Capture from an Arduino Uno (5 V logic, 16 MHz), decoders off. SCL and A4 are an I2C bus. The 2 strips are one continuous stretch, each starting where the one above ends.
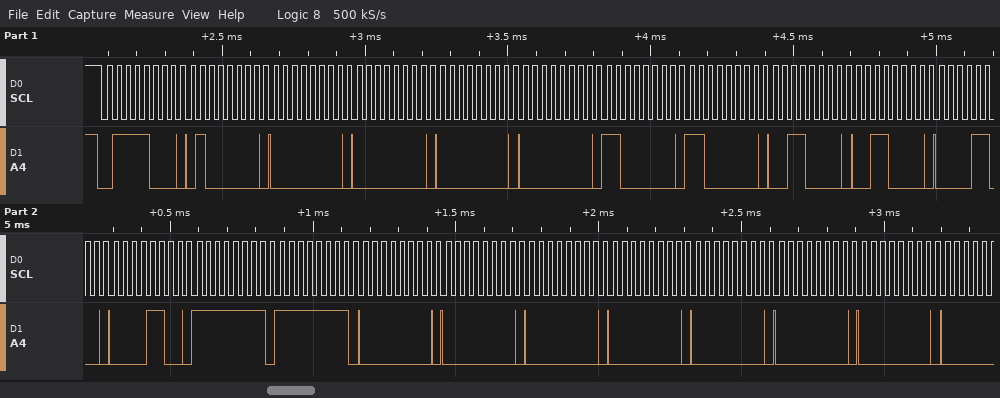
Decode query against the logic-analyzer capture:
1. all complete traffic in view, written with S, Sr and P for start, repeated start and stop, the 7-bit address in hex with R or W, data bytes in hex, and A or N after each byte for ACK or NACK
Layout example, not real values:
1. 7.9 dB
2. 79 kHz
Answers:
1. S 3CW A 40 A 00 A 00 A 00 A 00 A C0 A C0 A 30 A 30 A 0C A 0C A FF A FF A 00 A 00 A 00 A 00 A 00 A 00 A 00 A
